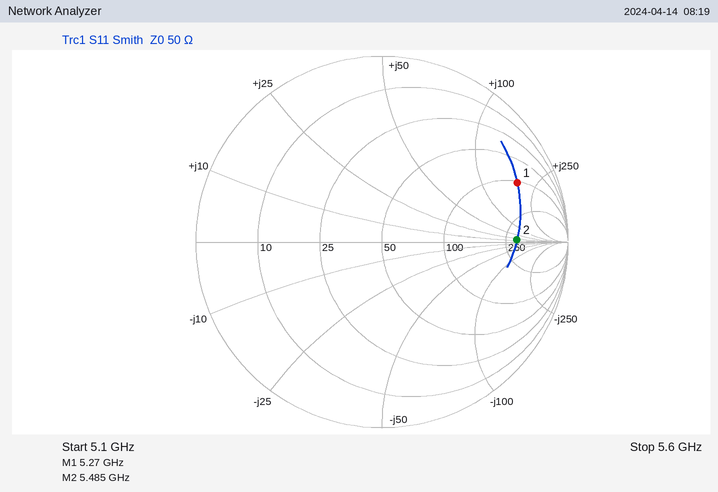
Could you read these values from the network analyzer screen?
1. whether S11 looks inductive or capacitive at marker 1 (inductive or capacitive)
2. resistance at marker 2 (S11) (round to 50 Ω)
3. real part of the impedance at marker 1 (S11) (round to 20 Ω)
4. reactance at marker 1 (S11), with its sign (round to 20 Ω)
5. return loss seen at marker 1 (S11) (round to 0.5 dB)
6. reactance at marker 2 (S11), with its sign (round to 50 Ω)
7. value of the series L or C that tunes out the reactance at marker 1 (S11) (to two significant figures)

inductive
300 Ω
100 Ω
+180 Ω
2.0 dB
0 Ω
170 fF
